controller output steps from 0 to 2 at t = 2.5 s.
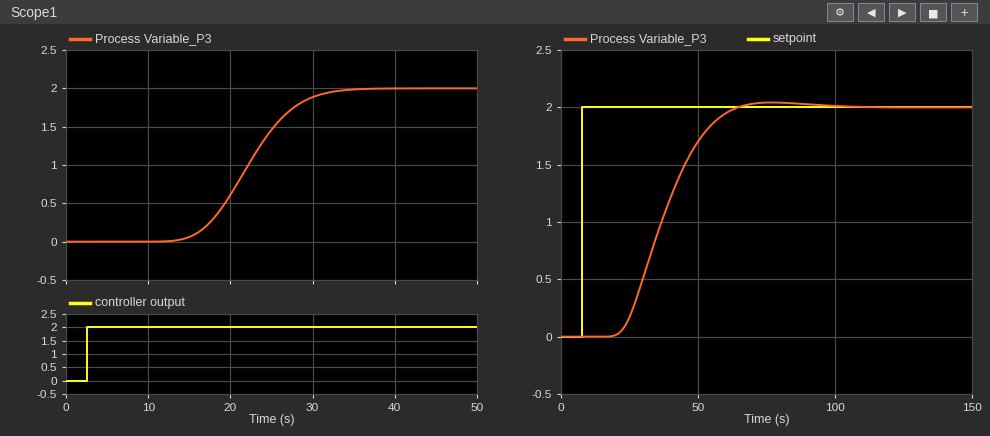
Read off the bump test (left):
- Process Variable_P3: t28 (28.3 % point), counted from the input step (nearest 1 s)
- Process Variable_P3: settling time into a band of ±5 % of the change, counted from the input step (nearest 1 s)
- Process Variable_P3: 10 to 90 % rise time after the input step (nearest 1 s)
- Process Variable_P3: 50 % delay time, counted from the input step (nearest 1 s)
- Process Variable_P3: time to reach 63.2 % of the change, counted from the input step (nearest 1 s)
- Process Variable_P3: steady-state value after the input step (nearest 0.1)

17 s
28 s
11 s
20 s
21 s
2.0
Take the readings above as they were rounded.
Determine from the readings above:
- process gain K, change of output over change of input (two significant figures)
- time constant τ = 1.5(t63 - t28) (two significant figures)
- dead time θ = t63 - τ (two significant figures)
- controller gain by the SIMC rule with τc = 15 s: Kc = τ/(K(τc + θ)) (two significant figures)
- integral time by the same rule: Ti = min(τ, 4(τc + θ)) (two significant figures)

1.0
6.0 s
15 s
0.20
6.0 s
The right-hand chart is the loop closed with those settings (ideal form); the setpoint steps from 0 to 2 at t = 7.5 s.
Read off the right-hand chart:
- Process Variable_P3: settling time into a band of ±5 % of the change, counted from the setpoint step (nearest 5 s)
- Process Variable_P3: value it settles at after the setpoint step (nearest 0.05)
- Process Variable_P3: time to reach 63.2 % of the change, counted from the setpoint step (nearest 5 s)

50 s
2.00
35 s
